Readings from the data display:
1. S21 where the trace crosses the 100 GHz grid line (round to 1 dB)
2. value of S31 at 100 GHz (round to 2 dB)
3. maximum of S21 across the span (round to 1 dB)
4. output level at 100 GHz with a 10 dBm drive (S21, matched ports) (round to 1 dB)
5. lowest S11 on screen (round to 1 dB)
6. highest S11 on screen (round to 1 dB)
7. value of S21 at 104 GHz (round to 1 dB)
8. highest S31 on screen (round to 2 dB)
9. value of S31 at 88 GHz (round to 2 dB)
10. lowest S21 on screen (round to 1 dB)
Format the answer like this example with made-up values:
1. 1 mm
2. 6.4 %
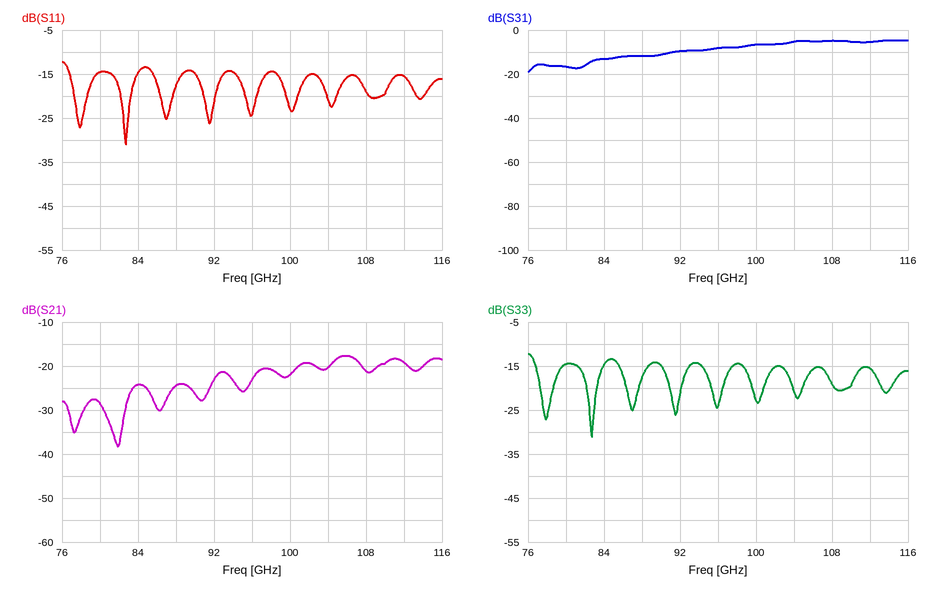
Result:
1. -22 dB
2. -6 dB
3. -18 dB
4. -12 dBm
5. -31 dB
6. -12 dB
7. -20 dB
8. -4 dB
9. -12 dB
10. -38 dB
